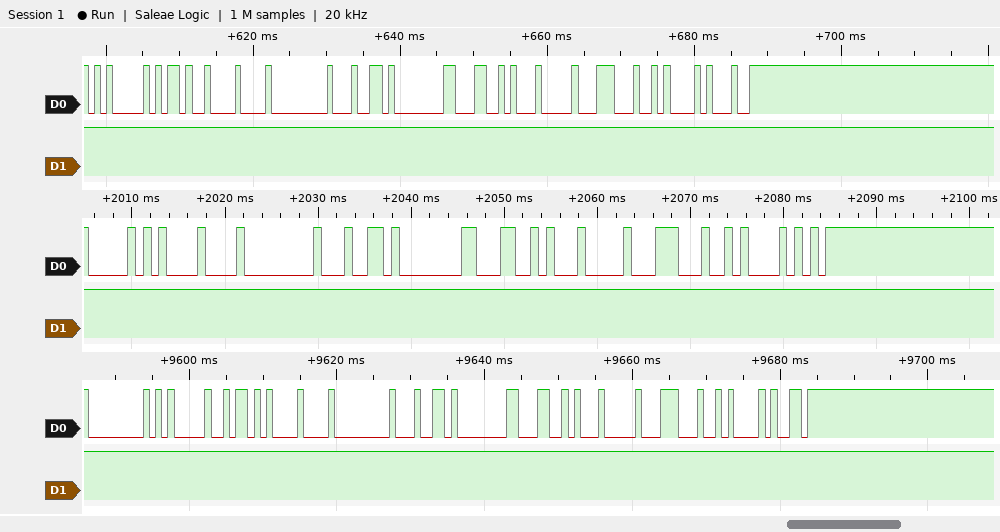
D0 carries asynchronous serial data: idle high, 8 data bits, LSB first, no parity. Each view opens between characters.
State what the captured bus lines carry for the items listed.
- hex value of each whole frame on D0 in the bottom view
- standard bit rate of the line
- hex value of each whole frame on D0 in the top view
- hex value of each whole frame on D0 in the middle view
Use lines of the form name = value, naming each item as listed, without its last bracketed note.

hex value of each whole frame on D0 in the bottom view = 00, 05, 5A, 08, 00, 64, 80, 4C, 04, 1C, 0A, D9
standard bit rate of the line = 1200 baud
hex value of each whole frame on D0 in the top view = 05, 2D, 08, 00, 64, 80, 4C, 04, 1C, 0A, 91
hex value of each whole frame on D0 in the middle view = 50, 08, 00, 64, 80, 4C, 04, 1C, 0A, F5
